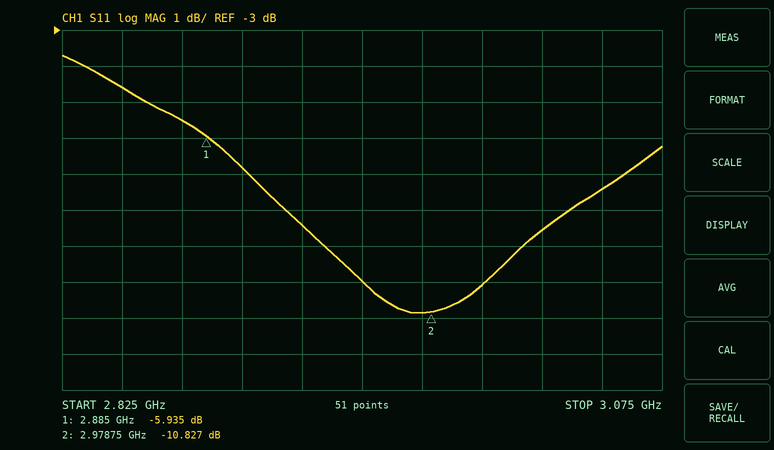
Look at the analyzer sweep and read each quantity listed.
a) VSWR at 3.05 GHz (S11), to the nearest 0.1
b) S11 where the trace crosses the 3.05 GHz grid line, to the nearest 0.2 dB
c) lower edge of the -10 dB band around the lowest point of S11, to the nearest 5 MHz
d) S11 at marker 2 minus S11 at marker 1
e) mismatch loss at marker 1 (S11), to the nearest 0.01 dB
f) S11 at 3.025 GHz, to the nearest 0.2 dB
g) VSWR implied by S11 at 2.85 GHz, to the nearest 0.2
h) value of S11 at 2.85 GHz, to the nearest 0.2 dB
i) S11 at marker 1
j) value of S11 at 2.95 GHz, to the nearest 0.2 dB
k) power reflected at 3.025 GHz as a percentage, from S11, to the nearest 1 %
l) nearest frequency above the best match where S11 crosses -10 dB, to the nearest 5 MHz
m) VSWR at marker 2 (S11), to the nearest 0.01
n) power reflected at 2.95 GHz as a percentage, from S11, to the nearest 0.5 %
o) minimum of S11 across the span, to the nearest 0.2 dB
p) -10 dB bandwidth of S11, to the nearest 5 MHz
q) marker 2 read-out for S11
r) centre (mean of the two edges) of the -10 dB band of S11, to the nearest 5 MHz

2.5
-7.4 dB
2.950 GHz
-4.892 dB
1.28 dB
-8.6 dB
3.8
-4.6 dB
-5.935 dB
-10.0 dB
14 %
3.000 GHz
1.81
10.0 %
-10.8 dB
50 MHz
-10.827 dB
2.975 GHz
